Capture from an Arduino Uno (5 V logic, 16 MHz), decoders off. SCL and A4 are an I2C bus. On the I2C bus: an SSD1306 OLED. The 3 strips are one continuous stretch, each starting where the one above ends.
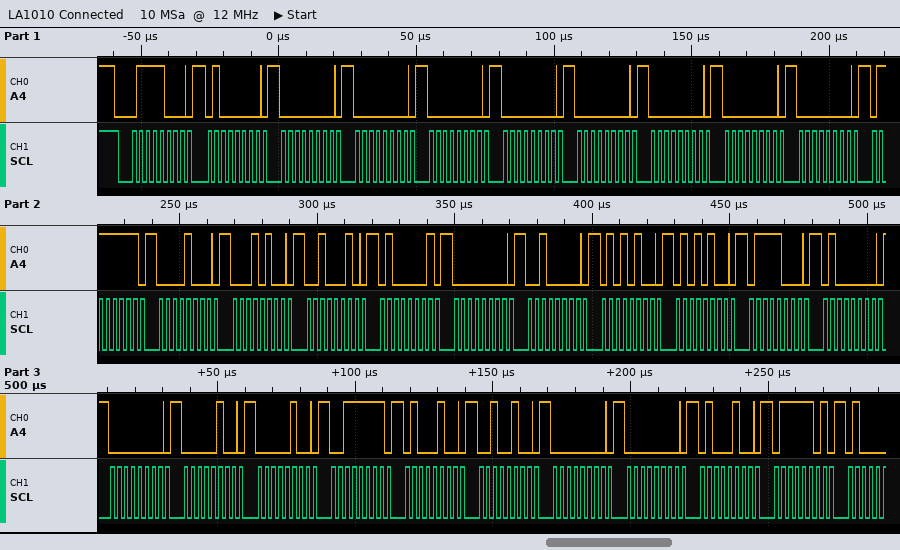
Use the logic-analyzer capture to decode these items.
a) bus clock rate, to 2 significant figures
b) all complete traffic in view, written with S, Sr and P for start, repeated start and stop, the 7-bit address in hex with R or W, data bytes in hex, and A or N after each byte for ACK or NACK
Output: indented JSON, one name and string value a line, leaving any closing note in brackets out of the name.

{
  "bus clock rate, to 2 significant figures": "400 kHz",
  "all complete traffic in view, written with S, Sr and P for start, repeated start and stop, the 7-bit address in hex with R or W, data bytes in hex, and A or N after each byte for ACK or NACK": "S 3CW A 40 A 00 A 00 A 00 A 00 A 00 A 00 A 00 A 00 A 7F A 08 A 14 A 22 A 41 A 00 A 20 A 54 A 54 A 78 A 40 A 00 A 04 A 04 A 3F A 44 A 24 A 00 A 00 A 44 A 7D A"
}
